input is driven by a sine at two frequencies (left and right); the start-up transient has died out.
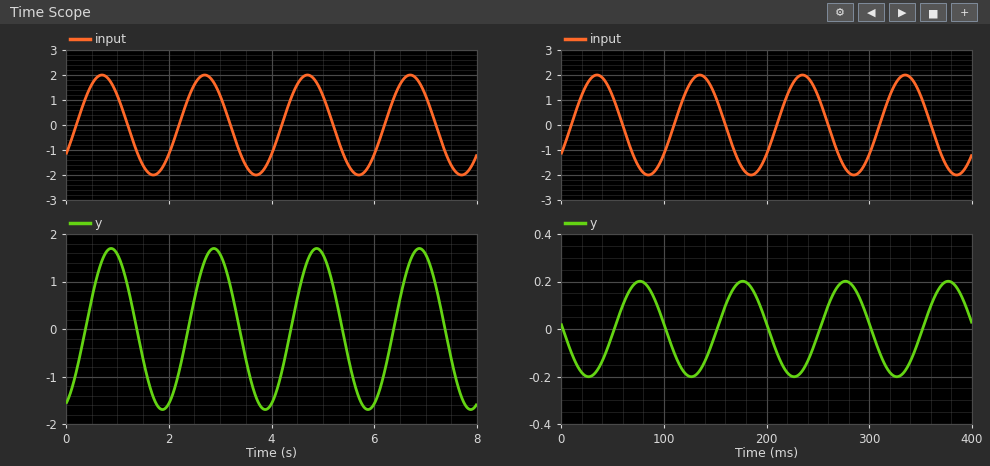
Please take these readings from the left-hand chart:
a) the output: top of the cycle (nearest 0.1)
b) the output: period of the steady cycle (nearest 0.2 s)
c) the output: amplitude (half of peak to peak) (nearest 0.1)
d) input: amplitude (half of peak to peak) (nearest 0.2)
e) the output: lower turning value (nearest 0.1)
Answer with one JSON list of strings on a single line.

["1.7", "2.0 s", "1.7", "2.0", "-1.7"]
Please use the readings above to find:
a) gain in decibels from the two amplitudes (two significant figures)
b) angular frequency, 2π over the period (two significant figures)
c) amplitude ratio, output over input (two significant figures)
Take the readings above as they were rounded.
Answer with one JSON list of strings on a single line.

["-1.4 dB", "3.1 rad/s", "0.85"]
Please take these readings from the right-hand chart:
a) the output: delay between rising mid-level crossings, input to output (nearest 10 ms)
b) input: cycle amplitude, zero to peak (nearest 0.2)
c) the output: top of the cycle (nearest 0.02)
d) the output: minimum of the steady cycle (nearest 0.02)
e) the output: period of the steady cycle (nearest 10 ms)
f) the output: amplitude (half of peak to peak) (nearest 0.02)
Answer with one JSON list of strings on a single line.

["40 ms", "2.0", "0.20", "-0.20", "100 ms", "0.20"]
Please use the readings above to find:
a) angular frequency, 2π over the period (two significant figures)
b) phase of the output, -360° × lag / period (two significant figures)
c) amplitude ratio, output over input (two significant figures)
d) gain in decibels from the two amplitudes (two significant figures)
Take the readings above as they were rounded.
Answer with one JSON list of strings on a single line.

["0.063 rad/ms", "-140°", "0.10", "-20 dB"]
